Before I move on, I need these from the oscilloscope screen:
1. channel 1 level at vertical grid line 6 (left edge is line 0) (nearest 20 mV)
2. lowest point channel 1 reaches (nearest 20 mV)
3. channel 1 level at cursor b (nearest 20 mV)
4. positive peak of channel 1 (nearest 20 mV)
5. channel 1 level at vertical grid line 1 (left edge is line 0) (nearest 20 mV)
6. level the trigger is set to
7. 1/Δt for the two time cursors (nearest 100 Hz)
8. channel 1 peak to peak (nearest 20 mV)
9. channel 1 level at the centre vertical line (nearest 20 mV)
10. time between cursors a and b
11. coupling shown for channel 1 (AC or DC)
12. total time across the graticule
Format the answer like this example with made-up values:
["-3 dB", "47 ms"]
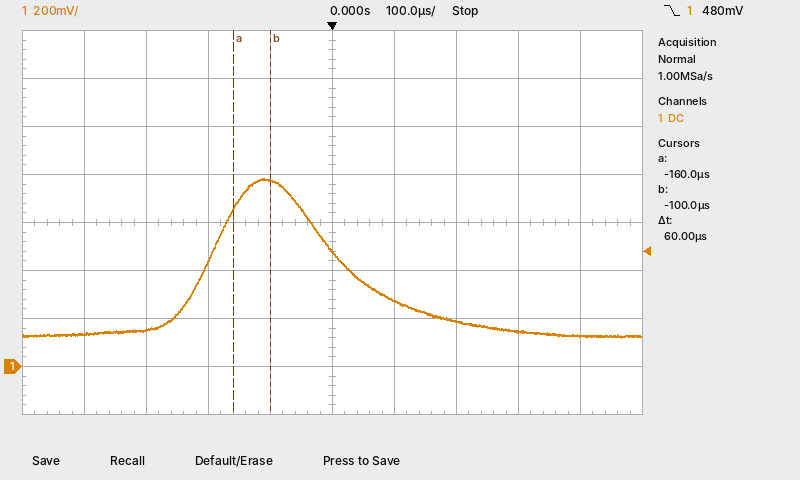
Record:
["280 mV", "120 mV", "780 mV", "780 mV", "140 mV", "480 mV", "16.7 kHz", "660 mV", "480 mV", "60 µs", "DC", "1 ms"]
